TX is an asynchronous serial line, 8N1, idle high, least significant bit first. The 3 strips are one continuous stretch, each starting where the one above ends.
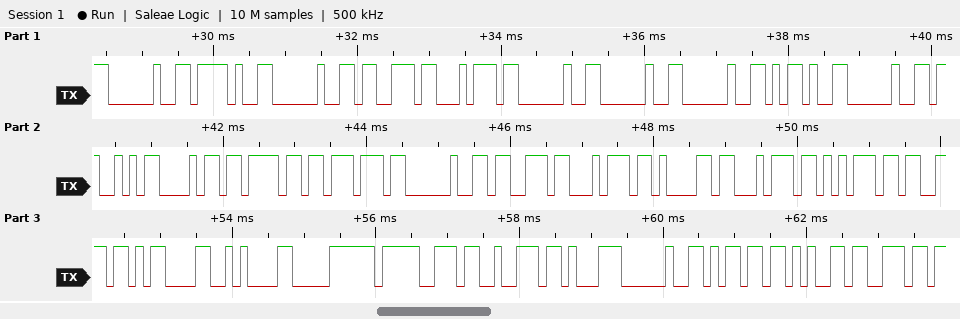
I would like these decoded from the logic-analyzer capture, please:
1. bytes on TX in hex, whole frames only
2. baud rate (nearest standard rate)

20 2F 20 73 74 20 20 20 2D 20 53 68 6F 77 20 73 74 61 74 75 73 0D 0A F0 9F 93 8B 20 6D 65 6E
9600 baud
